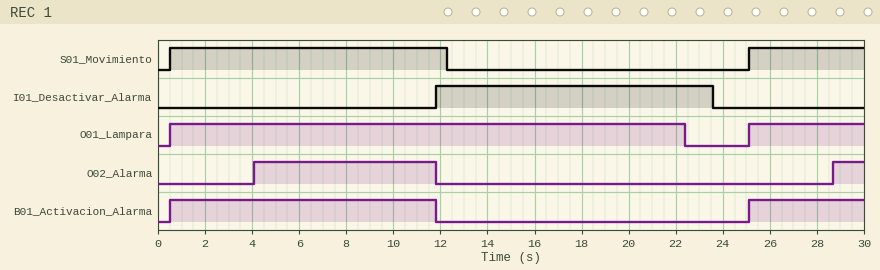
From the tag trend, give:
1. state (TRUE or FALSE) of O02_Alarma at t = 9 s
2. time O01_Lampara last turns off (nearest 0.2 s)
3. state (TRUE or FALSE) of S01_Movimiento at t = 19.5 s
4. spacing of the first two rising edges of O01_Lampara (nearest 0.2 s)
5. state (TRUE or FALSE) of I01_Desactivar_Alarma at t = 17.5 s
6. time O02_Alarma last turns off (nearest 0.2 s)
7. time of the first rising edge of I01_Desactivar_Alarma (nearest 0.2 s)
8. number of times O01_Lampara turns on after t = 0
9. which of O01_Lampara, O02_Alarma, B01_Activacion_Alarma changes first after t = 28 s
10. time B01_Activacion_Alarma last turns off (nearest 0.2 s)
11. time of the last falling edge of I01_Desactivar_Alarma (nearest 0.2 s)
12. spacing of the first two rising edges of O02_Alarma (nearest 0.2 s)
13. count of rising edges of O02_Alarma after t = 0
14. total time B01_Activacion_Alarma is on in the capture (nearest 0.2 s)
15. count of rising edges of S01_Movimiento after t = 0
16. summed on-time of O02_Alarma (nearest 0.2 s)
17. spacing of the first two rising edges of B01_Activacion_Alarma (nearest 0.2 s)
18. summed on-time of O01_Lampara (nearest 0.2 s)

TRUE
22.4 s
FALSE
24.6 s
TRUE
11.8 s
11.8 s
2
O02_Alarma
11.8 s
23.6 s
24.6 s
2
16.2 s
2
9.0 s
24.6 s
26.8 s
